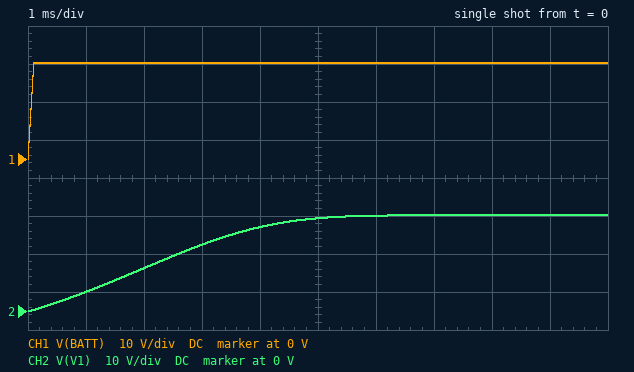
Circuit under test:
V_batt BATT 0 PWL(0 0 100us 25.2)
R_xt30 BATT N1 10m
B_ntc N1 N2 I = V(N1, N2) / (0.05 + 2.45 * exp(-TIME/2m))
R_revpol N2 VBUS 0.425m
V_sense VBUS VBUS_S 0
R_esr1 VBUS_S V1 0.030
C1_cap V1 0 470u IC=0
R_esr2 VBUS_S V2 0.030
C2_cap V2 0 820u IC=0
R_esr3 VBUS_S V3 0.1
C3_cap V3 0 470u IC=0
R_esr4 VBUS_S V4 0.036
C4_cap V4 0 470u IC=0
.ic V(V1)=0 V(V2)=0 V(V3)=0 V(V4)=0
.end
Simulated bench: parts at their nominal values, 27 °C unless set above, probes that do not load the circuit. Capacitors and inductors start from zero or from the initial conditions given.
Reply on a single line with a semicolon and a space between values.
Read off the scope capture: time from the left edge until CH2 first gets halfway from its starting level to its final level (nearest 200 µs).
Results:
2.2 ms
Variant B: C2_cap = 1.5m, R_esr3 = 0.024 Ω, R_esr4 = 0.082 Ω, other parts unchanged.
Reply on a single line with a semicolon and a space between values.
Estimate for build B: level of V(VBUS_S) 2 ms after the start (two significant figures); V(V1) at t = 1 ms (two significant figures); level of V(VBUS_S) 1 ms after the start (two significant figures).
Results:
9.3 V; 4.0 V; 4.1 V
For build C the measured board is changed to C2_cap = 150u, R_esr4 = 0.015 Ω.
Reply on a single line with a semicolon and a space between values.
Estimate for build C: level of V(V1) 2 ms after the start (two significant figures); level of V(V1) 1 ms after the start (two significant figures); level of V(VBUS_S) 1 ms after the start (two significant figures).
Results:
14 V; 6.8 V; 6.9 V
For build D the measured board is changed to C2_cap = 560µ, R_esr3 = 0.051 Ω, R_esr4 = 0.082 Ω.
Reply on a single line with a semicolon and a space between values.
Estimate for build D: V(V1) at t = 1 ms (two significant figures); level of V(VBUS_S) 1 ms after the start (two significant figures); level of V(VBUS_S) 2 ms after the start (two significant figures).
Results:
5.6 V; 5.7 V; 12 V
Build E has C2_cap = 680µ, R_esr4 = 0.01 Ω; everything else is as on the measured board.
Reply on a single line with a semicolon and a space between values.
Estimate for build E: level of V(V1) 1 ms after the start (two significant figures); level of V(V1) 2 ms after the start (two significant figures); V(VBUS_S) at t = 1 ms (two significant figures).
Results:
5.3 V; 12 V; 5.4 V
